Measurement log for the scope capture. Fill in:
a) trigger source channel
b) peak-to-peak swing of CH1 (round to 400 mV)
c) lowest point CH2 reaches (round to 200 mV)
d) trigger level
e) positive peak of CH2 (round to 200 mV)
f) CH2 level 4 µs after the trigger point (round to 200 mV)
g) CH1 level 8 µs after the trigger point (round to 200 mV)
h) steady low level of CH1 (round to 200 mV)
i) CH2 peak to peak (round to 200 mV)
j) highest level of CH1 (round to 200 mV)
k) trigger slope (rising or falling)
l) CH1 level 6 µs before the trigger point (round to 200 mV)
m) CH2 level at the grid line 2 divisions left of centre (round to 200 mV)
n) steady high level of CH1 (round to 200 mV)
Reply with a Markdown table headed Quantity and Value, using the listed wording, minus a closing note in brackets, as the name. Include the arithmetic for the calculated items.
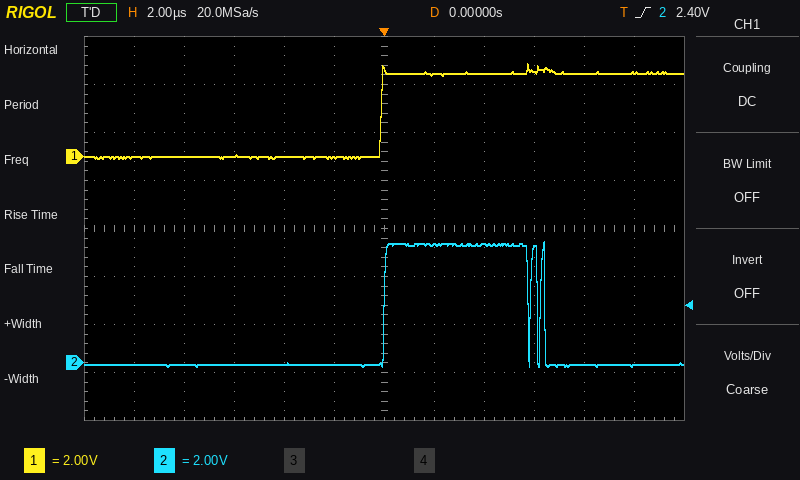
| Quantity | Value |
|---|---|
| trigger source channel | CH2 |
| peak-to-peak swing of CH1 | 4.0 V |
| lowest point CH2 reaches | -200 mV |
| trigger level | 2.40 V |
| positive peak of CH2 | 5.0 V |
| CH2 level 4 µs after the trigger point | 5.0 V |
| CH1 level 8 µs after the trigger point | 3.4 V |
| steady low level of CH1 | 0.0 V |
| CH2 peak to peak | 5.0 V − (-200 mV) = 5.2 V |
| highest level of CH1 | 3.8 V |
| trigger slope | rising |
| CH1 level 6 µs before the trigger point | 0.0 V |
| CH2 level at the grid line 2 divisions left of centre | 0.0 V |
| steady high level of CH1 | 3.4 V |
